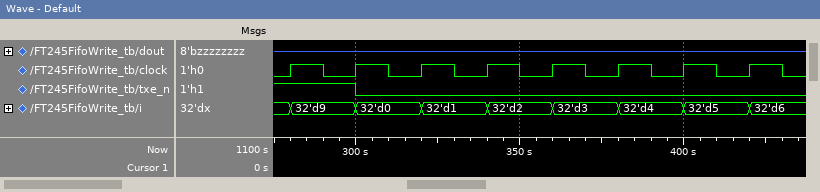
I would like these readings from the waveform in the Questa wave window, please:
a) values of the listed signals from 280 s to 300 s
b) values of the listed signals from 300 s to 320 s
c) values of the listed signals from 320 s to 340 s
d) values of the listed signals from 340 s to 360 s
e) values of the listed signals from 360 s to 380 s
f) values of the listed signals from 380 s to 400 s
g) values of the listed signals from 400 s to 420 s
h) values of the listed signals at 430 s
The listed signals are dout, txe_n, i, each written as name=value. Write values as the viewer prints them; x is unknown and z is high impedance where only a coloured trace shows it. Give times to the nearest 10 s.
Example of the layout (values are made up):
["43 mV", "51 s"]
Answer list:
["dout=z, txe_n=1, i=32'd9", "dout=z, txe_n=0, i=32'd0", "dout=z, txe_n=0, i=32'd1", "dout=z, txe_n=0, i=32'd2", "dout=z, txe_n=0, i=32'd3", "dout=z, txe_n=0, i=32'd4", "dout=z, txe_n=0, i=32'd5", "dout=z, txe_n=0, i=32'd6"]
